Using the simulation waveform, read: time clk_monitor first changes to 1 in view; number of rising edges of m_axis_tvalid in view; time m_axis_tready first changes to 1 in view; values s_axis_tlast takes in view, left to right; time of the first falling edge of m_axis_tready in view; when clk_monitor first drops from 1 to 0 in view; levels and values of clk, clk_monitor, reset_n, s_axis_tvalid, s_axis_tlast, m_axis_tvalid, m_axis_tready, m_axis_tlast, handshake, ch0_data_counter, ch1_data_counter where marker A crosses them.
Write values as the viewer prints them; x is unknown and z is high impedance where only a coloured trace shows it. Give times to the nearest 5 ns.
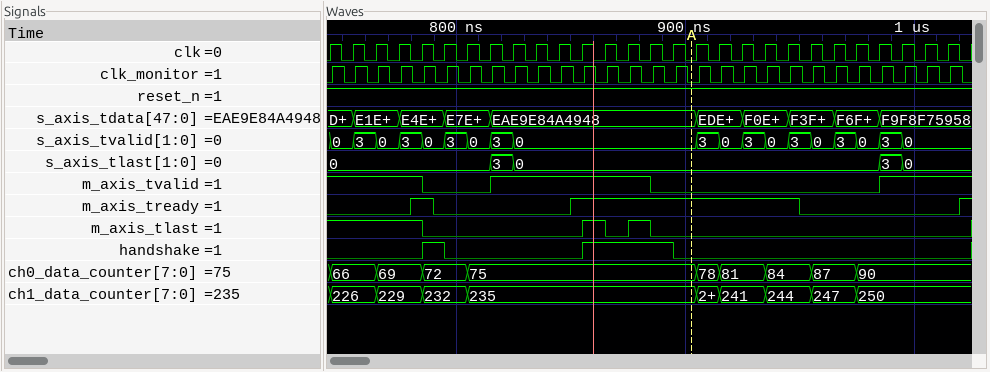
745 ns
2
780 ns
0, 3, 0, 3, 0
790 ns
750 ns
clk=0, clk_monitor=0, reset_n=1, s_axis_tvalid=0, s_axis_tlast=0, m_axis_tvalid=0, m_axis_tready=1, m_axis_tlast=0, handshake=0, ch0_data_counter=75, ch1_data_counter=235
